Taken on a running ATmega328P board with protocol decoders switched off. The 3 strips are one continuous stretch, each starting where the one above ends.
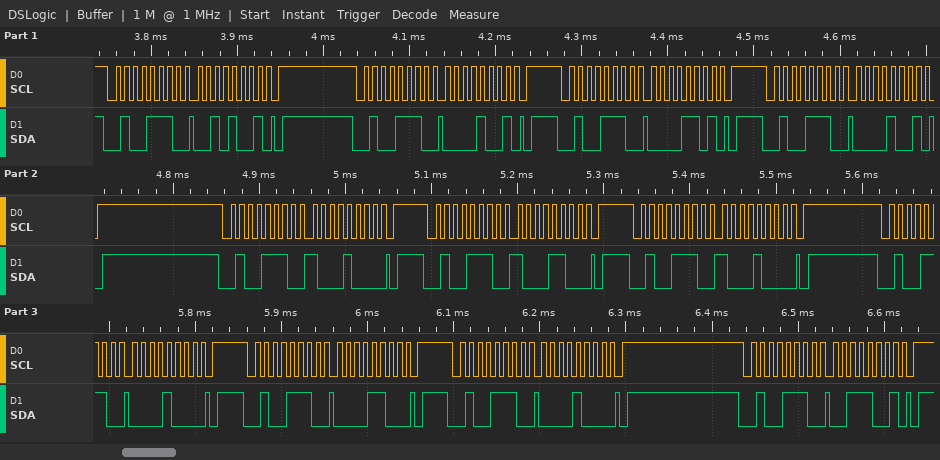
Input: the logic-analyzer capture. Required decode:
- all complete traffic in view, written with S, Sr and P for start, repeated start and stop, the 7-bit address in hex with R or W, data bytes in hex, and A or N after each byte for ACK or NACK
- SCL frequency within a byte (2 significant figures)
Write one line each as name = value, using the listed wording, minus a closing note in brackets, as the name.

all complete traffic in view, written with S, Sr and P for start, repeated start and stop, the 7-bit address in hex with R or W, data bytes in hex, and A or N after each byte for ACK or NACK = S 27W A 29 A P S 27W A 09 A P S 27W A 0D A P S 27W A 09 A P S 27W A 88 A P S 27W A 8C A P S 27W A 88 A P S 27W A 08 A P S 27W A 0C A P S 27W A 08 A P S 27W A 39 A P
SCL frequency within a byte = 100 kHz
